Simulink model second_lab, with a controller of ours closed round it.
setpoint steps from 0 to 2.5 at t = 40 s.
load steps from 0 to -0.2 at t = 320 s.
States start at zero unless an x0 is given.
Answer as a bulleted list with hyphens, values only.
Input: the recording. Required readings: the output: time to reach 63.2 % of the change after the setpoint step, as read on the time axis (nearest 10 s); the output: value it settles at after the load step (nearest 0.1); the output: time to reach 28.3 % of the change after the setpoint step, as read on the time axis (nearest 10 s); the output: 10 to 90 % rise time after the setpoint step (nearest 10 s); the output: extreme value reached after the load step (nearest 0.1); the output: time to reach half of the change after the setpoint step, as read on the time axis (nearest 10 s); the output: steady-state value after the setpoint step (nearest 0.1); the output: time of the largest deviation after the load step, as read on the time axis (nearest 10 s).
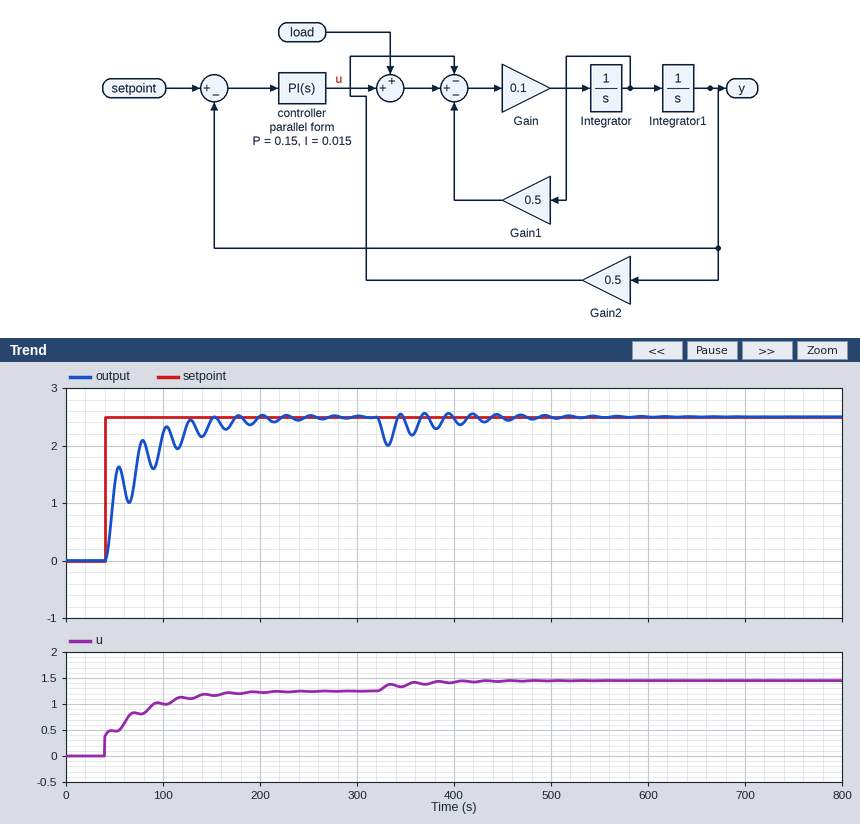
- 50 s
- 2.5
- 50 s
- 60 s
- 2.0
- 50 s
- 2.5
- 330 s
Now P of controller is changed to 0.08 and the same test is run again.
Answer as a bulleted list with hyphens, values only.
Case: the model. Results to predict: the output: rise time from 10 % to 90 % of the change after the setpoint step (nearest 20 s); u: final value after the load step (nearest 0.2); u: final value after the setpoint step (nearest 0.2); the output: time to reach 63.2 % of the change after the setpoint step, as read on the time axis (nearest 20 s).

- 60 s
- 1.4
- 1.2
- 80 s
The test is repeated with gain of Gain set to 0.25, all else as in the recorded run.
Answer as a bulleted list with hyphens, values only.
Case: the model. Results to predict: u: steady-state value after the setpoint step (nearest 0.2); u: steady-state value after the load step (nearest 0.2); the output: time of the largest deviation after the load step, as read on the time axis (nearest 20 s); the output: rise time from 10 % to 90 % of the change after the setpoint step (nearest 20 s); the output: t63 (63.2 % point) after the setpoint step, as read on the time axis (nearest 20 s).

- 1.2
- 1.4
- 320 s
- 80 s
- 60 s
